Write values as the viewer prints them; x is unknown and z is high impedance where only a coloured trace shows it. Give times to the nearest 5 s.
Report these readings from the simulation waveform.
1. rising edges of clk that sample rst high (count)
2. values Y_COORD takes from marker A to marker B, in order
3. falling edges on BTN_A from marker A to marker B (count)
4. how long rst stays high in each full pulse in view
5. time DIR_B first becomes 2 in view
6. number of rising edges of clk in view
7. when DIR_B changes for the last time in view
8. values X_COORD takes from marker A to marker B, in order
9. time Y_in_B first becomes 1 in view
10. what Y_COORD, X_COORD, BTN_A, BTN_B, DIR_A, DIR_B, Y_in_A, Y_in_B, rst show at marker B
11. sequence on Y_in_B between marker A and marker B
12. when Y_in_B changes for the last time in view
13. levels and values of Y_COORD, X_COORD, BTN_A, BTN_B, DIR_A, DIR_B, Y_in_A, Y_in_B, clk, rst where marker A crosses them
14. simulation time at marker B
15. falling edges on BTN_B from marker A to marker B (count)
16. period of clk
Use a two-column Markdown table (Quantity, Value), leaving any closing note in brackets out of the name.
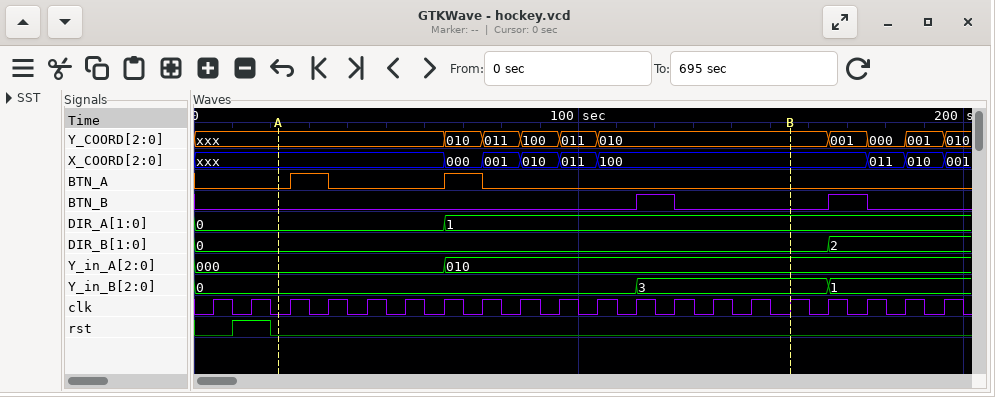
| Quantity | Value |
|---|---|
| rising edges of clk that sample rst high | 1 |
| values Y_COORD takes from marker A to marker B, in order | xxx, 010, 011, 100, 011, 010 |
| falling edges on BTN_A from marker A to marker B | 2 |
| how long rst stays high in each full pulse in view | 10 s |
| time DIR_B first becomes 2 in view | 165 s |
| number of rising edges of clk in view | 20 |
| when DIR_B changes for the last time in view | 165 s |
| values X_COORD takes from marker A to marker B, in order | xxx, 000, 001, 010, 011, 100 |
| time Y_in_B first becomes 1 in view | 165 s |
| what Y_COORD, X_COORD, BTN_A, BTN_B, DIR_A, DIR_B, Y_in_A, Y_in_B, rst show at marker B | Y_COORD=010, X_COORD=100, BTN_A=0, BTN_B=0, DIR_A=1, DIR_B=0, Y_in_A=010, Y_in_B=3, rst=0 |
| sequence on Y_in_B between marker A and marker B | 0, 3 |
| when Y_in_B changes for the last time in view | 165 s |
| levels and values of Y_COORD, X_COORD, BTN_A, BTN_B, DIR_A, DIR_B, Y_in_A, Y_in_B, clk, rst where marker A crosses them | Y_COORD=xxx, X_COORD=xxx, BTN_A=0, BTN_B=0, DIR_A=0, DIR_B=0, Y_in_A=000, Y_in_B=0, clk=0, rst=0 |
| simulation time at marker B | 155 s |
| falling edges on BTN_B from marker A to marker B | 1 |
| period of clk | 10 s |
